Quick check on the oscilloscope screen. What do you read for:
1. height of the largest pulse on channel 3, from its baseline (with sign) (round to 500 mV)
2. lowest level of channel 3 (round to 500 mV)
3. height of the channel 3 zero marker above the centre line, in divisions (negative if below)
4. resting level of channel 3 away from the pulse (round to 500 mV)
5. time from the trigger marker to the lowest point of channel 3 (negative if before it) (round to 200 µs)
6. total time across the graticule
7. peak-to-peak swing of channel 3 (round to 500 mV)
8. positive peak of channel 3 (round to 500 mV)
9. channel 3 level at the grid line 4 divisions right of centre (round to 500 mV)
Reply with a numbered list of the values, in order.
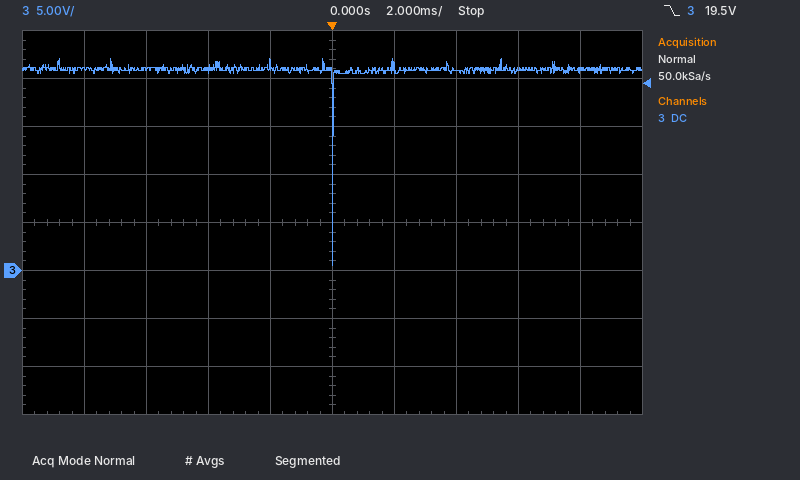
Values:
1. -20.5 V
2. 500 mV
3. -1.0 div
4. 21.0 V
5. 0.0 ms
6. 20 ms
7. 21.5 V
8. 22.0 V
9. 21.0 V
